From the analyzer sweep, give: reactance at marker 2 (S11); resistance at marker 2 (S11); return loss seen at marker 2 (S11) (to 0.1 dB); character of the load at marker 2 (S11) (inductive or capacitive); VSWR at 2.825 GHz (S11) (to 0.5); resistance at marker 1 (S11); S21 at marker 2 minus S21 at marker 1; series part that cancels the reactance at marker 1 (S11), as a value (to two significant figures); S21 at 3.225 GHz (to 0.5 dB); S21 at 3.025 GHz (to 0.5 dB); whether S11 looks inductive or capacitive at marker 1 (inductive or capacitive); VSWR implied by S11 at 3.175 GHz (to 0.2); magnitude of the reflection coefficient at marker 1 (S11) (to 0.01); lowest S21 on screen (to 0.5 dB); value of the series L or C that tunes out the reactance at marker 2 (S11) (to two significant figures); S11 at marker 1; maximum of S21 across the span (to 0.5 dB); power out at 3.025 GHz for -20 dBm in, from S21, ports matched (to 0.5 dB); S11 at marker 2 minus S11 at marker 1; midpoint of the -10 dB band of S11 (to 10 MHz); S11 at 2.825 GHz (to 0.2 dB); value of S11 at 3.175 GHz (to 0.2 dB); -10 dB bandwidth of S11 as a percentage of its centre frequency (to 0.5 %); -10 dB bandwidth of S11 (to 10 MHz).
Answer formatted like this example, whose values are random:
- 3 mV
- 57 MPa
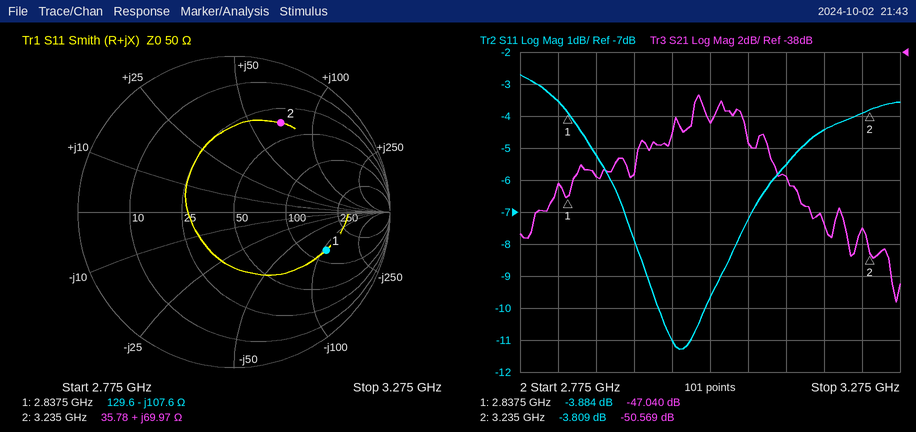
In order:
- +69.97 Ω
- 35.78 Ω
- 3.8 dB
- inductive
- 5.0
- 129.6 Ω
- -3.529 dB
- 6.0 nH
- -49.0 dB
- -42.5 dB
- capacitive
- 4.0
- 0.64
- -53.5 dB
- 700 fF
- -3.884 dB
- -40.5 dB
- -62.5 dBm
- 0.075 dB
- 2.99 GHz
- -3.6 dB
- -4.4 dB
- 2.0 %
- 60 MHz
